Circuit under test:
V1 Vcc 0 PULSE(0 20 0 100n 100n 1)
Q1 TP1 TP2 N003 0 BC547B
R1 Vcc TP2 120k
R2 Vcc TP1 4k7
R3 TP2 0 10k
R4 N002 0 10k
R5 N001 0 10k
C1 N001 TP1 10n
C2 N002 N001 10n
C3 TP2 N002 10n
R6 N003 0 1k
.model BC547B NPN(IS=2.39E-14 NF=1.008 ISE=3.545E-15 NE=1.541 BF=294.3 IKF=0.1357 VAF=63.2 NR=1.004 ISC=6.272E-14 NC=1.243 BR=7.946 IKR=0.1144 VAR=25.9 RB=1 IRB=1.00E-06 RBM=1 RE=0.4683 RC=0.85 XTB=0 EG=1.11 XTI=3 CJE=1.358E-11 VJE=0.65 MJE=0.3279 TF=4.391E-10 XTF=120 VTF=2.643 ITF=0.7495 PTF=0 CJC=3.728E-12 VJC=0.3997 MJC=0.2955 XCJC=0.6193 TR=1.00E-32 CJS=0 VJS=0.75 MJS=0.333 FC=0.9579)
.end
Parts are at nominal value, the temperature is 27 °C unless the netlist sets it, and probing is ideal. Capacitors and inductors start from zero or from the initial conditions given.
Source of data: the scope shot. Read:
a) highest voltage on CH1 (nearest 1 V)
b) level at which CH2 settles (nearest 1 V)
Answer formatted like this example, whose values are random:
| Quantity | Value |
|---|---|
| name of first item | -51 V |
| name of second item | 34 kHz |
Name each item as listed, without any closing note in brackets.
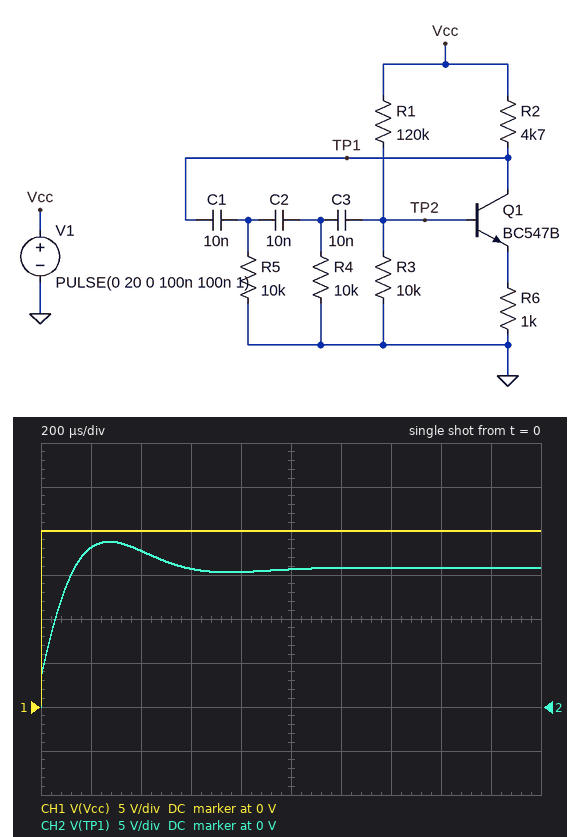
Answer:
| Quantity | Value |
|---|---|
| highest voltage on CH1 | 20 V |
| level at which CH2 settles | 16 V |
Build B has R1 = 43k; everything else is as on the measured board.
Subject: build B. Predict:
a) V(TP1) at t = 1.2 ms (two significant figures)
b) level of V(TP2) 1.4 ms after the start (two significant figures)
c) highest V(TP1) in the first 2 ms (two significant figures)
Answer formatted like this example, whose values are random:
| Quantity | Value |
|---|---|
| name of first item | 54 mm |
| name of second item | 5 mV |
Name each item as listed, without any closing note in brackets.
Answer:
| Quantity | Value |
|---|---|
| V(TP1) at t = 1.2 ms | 5.9 V |
| level of V(TP2) 1.4 ms after the start | 3.7 V |
| highest V(TP1) in the first 2 ms | 9.8 V |
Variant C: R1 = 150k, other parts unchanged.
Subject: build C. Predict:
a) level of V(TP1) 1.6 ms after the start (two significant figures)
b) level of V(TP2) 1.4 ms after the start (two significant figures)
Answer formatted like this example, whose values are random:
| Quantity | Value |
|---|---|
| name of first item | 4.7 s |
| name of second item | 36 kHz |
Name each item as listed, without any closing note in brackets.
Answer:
| Quantity | Value |
|---|---|
| level of V(TP1) 1.6 ms after the start | 17 V |
| level of V(TP2) 1.4 ms after the start | 1.2 V |
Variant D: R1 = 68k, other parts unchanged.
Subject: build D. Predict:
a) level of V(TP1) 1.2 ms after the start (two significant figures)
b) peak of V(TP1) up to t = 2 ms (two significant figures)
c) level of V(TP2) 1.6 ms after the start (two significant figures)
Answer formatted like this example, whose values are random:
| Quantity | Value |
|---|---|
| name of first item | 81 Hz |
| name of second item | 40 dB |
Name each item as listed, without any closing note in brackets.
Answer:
| Quantity | Value |
|---|---|
| level of V(TP1) 1.2 ms after the start | 11 V |
| peak of V(TP1) up to t = 2 ms | 15 V |
| level of V(TP2) 1.6 ms after the start | 2.5 V |
